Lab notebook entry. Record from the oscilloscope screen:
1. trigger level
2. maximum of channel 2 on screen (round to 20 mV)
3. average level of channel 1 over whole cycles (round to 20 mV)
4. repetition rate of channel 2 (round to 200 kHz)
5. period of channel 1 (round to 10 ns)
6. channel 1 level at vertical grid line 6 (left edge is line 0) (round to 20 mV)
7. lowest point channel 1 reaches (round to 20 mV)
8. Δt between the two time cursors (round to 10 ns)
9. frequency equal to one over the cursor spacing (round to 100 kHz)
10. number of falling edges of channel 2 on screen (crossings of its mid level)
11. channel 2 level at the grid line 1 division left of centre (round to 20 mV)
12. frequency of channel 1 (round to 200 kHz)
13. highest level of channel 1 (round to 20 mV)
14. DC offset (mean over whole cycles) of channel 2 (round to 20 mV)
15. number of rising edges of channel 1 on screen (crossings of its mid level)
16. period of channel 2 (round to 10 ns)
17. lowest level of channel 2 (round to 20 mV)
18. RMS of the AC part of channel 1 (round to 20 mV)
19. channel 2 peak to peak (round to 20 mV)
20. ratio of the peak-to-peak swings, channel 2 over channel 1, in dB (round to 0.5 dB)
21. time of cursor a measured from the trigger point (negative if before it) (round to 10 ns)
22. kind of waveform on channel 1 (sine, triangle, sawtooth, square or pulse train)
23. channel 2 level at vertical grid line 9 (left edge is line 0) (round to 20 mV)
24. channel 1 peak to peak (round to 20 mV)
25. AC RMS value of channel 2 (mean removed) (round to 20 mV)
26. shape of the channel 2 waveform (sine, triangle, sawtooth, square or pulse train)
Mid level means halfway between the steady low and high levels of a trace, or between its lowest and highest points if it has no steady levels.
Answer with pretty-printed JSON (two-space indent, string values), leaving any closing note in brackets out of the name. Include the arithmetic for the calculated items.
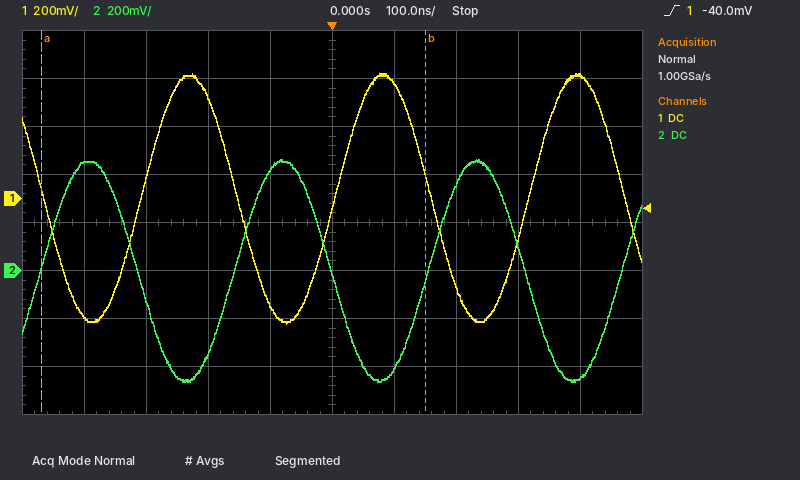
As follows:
{
  "trigger level": "-40.0 mV",
  "maximum of channel 2 on screen": "460 mV",
  "average level of channel 1 over whole cycles": "(520 mV + (-520 mV)) / 2 ≈ 0 mV",
  "repetition rate of channel 2": "1 / 310 ns ≈ 3.2 MHz",
  "period of channel 1": "310 ns",
  "channel 1 level at vertical grid line 6 (left edge is line 0)": "480 mV",
  "lowest point channel 1 reaches": "-520 mV",
  "Δt between the two time cursors": "620 ns",
  "frequency equal to one over the cursor spacing": "1 / 620 ns ≈ 1.6 MHz",
  "number of falling edges of channel 2 on screen": "3",
  "channel 2 level at the grid line 1 division left of centre": "420 mV",
  "frequency of channel 1": "1 / 310 ns ≈ 3.2 MHz",
  "highest level of channel 1": "520 mV",
  "DC offset (mean over whole cycles) of channel 2": "(460 mV + (-460 mV)) / 2 ≈ 0 mV",
  "number of rising edges of channel 1 on screen": "3",
  "period of channel 2": "310 ns",
  "lowest level of channel 2": "-460 mV",
  "RMS of the AC part of channel 1": "1.04 V / (2√2) ≈ 368 mV, so 360 mV to the nearest 20 mV",
  "channel 2 peak to peak": "460 mV − (-460 mV) = 920 mV",
  "ratio of the peak-to-peak swings, channel 2 over channel 1, in dB": "20 log10(920 mV / 1.04 V) ≈ -1.06 dB, so -1.0 dB to the nearest 0.5 dB",
  "time of cursor a measured from the trigger point (negative if before it)": "-470 ns",
  "kind of waveform on channel 1": "sine",
  "channel 2 level at vertical grid line 9 (left edge is line 0)": "-440 mV",
  "channel 1 peak to peak": "520 mV − (-520 mV) = 1.04 V",
  "AC RMS value of channel 2 (mean removed)": "920 mV / (2√2) ≈ 325 mV, so 320 mV to the nearest 20 mV",
  "shape of the channel 2 waveform": "sine"
}
